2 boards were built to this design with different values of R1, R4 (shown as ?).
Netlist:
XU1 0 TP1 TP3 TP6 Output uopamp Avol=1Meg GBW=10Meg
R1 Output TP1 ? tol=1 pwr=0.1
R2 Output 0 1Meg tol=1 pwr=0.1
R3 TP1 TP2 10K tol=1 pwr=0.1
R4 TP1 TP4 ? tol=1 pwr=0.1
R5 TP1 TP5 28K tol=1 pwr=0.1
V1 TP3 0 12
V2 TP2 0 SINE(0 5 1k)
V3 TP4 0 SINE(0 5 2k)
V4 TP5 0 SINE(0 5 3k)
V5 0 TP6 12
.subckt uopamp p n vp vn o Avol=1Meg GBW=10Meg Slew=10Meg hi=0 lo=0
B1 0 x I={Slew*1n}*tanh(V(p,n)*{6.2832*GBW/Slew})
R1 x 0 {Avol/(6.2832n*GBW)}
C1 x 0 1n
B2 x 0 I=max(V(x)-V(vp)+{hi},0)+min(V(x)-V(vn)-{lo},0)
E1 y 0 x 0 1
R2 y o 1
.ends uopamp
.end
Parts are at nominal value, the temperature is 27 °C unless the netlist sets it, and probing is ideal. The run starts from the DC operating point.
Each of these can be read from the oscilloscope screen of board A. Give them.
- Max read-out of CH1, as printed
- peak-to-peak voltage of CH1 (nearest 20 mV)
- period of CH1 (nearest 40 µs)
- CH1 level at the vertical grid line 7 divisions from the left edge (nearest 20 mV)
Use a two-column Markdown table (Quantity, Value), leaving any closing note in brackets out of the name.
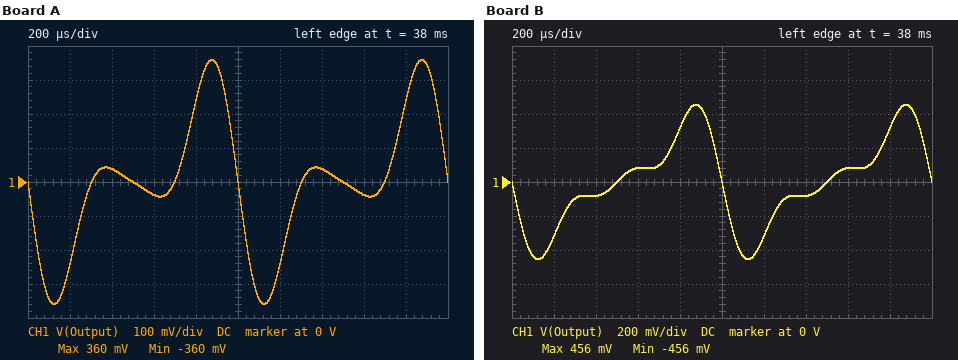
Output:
| Quantity | Value |
|---|---|
| Max read-out of CH1, as printed | 360 mV |
| peak-to-peak voltage of CH1 | 720 mV |
| period of CH1 | 1.00 ms |
| CH1 level at the vertical grid line 7 divisions from the left edge | 40 mV |
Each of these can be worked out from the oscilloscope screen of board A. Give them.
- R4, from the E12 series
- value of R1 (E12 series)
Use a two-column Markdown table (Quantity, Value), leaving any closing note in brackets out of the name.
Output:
| Quantity | Value |
|---|---|
| R4, from the E12 series | 8.2 kΩ |
| value of R1 | 330 Ω |
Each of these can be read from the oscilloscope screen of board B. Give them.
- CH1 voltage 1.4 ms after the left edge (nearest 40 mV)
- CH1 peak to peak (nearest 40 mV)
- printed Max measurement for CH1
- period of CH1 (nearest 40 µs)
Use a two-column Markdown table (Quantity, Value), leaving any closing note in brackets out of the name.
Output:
| Quantity | Value |
|---|---|
| CH1 voltage 1.4 ms after the left edge | -80 mV |
| CH1 peak to peak | 920 mV |
| printed Max measurement for CH1 | 456 mV |
| period of CH1 | 1.00 ms |
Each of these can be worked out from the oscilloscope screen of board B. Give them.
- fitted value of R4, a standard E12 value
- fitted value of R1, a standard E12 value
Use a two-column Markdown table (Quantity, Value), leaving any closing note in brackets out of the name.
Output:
| Quantity | Value |
|---|---|
| fitted value of R4, a standard E12 value | 15 kΩ |
| fitted value of R1, a standard E12 value | 560 Ω |
